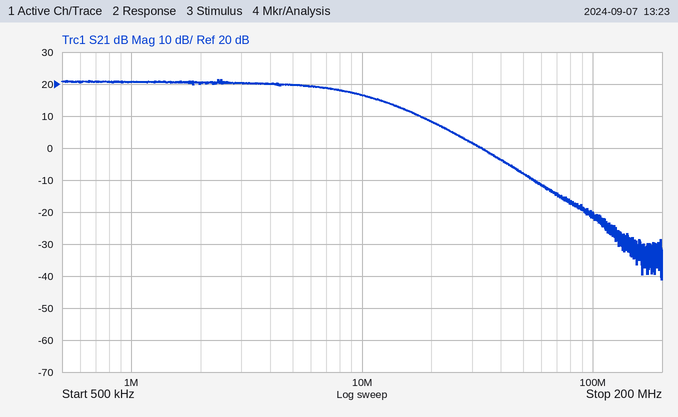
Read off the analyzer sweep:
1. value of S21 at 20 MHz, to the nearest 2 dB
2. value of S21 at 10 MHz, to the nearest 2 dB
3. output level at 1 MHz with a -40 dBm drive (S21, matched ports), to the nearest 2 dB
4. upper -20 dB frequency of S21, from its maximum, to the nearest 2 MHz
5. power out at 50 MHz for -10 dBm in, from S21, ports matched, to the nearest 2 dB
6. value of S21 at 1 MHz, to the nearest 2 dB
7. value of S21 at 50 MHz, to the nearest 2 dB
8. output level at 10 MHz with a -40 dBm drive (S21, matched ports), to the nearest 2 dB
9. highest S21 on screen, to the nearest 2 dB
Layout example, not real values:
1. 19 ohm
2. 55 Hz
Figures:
1. 8 dB
2. 16 dB
3. -20 dBm
4. 30 MHz
5. -18 dBm
6. 20 dB
7. -8 dB
8. -24 dBm
9. 22 dB
